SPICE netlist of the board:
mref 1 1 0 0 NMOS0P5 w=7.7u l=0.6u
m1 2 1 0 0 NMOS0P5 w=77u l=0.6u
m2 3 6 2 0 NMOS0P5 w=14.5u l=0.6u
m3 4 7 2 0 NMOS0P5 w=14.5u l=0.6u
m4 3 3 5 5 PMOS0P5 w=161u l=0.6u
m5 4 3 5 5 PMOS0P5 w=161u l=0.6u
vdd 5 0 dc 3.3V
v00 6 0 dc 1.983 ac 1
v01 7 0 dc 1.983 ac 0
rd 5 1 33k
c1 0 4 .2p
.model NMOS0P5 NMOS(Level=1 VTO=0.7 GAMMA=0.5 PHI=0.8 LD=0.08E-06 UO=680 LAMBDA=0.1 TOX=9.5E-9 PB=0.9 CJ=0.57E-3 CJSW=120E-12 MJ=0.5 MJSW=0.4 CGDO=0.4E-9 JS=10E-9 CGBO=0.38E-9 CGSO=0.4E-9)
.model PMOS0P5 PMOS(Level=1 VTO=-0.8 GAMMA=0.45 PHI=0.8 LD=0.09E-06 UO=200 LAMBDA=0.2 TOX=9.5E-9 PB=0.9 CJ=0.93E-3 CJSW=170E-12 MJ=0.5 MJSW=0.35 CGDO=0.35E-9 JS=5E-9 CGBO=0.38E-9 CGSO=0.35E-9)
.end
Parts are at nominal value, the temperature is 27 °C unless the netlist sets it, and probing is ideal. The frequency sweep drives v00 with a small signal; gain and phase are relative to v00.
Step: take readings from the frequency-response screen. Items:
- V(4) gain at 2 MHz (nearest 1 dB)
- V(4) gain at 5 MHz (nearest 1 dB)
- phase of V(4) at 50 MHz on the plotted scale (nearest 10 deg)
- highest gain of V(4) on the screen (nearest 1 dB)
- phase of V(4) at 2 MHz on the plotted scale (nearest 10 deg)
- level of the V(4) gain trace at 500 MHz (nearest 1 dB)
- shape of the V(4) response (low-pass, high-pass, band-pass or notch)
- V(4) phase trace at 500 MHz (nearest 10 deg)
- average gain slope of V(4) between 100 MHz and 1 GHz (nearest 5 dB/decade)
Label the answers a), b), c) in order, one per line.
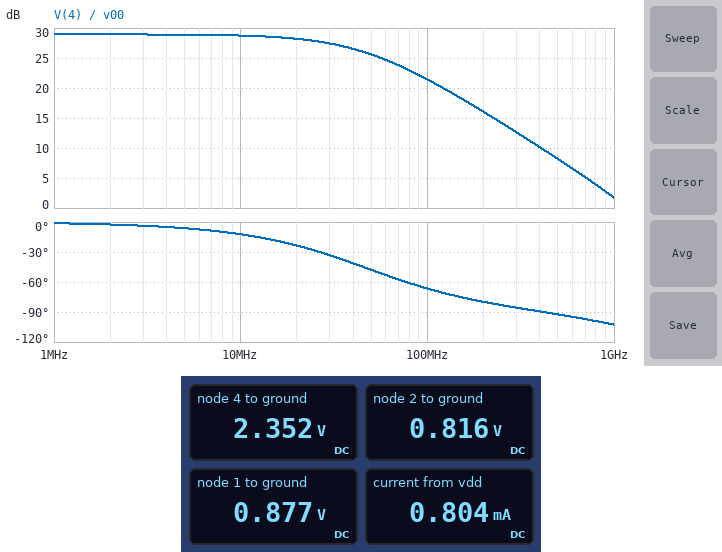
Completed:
a) 29 dB
b) 29 dB
c) -50 deg
d) 29 dB
e) 0 deg
f) 8 dB
g) low-pass
h) -90 deg
i) -20 dB/decade
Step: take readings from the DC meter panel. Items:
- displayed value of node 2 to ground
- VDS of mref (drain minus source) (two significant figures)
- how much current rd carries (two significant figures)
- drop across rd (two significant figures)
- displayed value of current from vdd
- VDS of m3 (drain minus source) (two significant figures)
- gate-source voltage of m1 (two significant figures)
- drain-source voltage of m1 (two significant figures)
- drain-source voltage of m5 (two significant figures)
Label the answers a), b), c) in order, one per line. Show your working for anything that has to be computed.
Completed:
a) 0.816 V
b) 877 mV = 880 mV
c) (3.3 V - 877 mV) / 33 kΩ = 73 µA
d) 3.3 V - 877 mV = 2.4 V
e) 0.804 mA
f) 2.352 V - 816 mV = 1.5 V
g) 877 mV = 880 mV
h) 816 mV = 820 mV
i) 2.352 V - 3.3 V = -950 mV
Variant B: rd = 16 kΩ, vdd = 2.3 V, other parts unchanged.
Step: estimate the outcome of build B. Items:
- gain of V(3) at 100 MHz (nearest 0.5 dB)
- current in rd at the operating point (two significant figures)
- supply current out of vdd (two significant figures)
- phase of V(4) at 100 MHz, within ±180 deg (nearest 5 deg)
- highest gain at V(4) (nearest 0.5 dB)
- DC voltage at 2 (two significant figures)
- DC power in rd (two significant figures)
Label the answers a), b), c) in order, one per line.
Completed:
a) -15.5 dB
b) 88 µA
c) 960 µA
d) -60 deg
e) 27.5 dB
f) 780 mV
g) 120 µW
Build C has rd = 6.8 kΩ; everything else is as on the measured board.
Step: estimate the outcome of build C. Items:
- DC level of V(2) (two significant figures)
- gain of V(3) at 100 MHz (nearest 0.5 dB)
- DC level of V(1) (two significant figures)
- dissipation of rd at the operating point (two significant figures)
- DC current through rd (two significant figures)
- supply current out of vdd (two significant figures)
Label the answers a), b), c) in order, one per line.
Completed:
a) 570 mV
b) -15.0 dB
c) 1.1 V
d) 730 µW
e) 330 µA
f) 3.5 mA
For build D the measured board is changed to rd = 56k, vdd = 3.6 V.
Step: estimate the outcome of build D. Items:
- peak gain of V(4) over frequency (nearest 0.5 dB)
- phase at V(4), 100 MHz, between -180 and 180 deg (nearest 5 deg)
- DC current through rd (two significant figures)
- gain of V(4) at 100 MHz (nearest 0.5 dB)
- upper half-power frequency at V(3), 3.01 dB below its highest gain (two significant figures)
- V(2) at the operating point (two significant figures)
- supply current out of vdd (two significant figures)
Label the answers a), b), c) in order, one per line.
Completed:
a) 31.0 dB
b) -75 deg
c) 49 µA
d) 20.5 dB
e) 2.1 GHz
f) 860 mV
g) 540 µA
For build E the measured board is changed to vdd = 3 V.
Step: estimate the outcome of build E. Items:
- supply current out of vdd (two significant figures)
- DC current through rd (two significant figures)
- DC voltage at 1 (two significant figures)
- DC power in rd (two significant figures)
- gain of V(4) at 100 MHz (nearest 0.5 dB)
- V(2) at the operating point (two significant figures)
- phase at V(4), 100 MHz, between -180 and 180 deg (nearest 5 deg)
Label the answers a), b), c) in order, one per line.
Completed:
a) 710 µA
b) 65 µA
c) 870 mV
d) 140 µW
e) 21.0 dB
f) 830 mV
g) -70 deg
